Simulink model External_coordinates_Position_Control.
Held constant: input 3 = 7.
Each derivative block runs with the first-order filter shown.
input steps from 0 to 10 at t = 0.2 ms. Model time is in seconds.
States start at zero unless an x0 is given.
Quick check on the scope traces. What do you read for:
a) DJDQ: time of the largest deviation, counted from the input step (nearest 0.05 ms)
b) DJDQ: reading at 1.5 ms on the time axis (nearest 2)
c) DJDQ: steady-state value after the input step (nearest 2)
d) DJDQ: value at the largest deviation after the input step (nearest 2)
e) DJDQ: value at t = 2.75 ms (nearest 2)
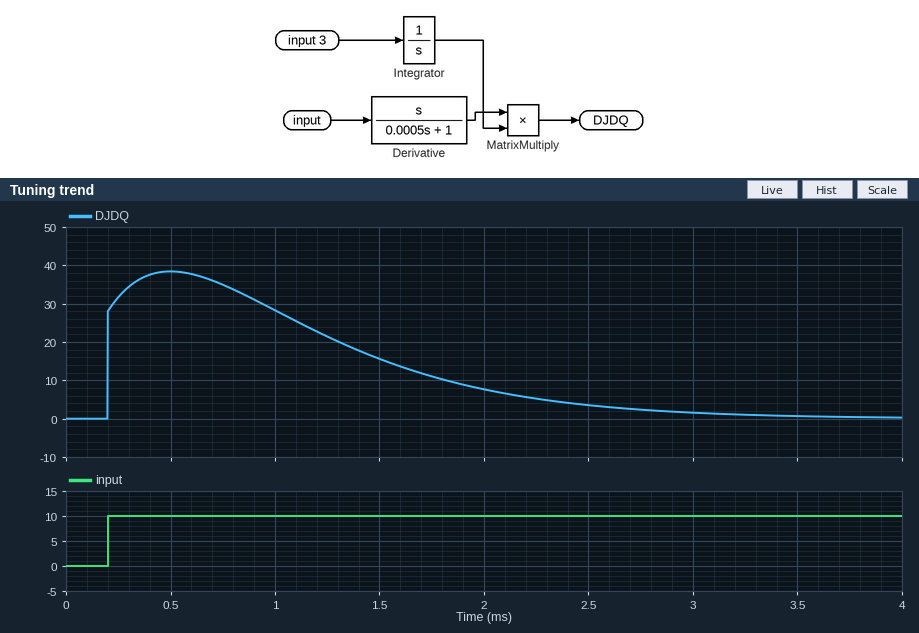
0.30 ms
16
0
38
2
